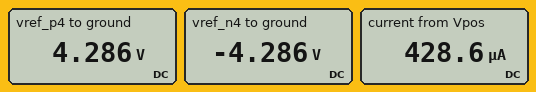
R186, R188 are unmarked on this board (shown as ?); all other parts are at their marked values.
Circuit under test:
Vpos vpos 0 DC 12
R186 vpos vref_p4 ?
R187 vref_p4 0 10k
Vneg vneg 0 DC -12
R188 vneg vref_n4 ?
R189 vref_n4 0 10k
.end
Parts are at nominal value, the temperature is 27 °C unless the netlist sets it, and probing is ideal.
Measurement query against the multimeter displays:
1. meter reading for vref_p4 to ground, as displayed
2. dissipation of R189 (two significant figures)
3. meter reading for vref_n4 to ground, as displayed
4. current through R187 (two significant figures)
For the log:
4.286 V
1.8 mW
-4.286 V
430 µA
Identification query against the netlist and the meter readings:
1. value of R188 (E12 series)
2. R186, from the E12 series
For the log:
18 kΩ
18 kΩ
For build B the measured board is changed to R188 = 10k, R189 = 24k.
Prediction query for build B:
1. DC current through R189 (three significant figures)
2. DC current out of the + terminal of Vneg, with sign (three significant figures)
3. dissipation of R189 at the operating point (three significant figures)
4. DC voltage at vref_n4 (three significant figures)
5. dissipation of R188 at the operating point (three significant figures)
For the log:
353 µA
-353 µA
2.99 mW
-8.47 V
1.25 mW
